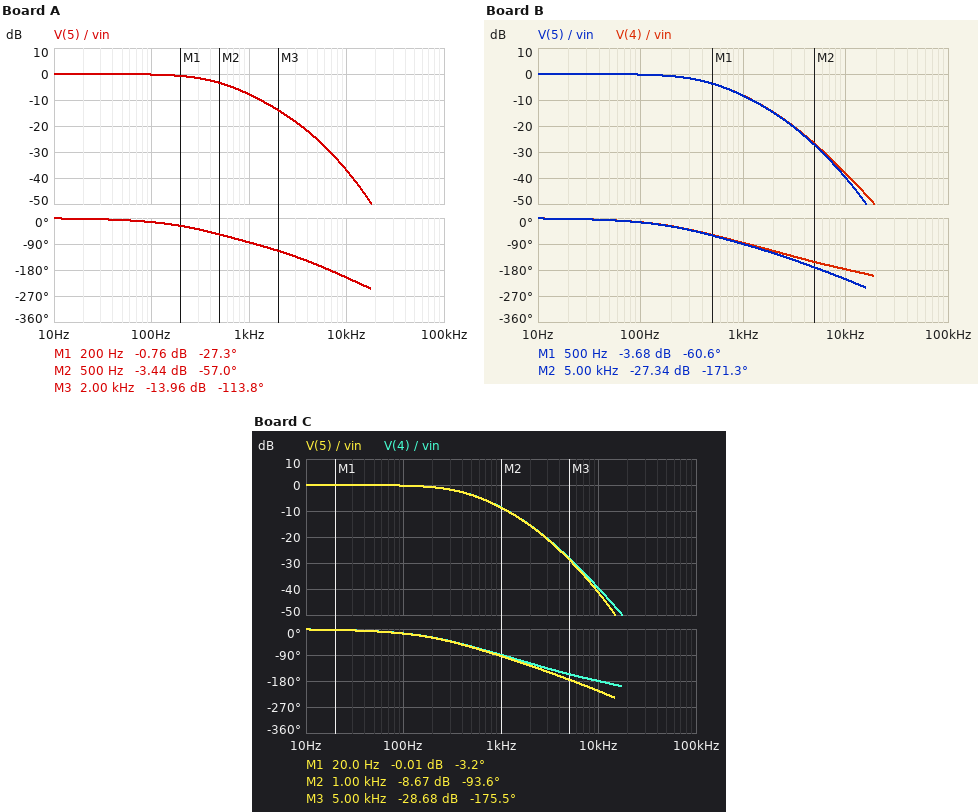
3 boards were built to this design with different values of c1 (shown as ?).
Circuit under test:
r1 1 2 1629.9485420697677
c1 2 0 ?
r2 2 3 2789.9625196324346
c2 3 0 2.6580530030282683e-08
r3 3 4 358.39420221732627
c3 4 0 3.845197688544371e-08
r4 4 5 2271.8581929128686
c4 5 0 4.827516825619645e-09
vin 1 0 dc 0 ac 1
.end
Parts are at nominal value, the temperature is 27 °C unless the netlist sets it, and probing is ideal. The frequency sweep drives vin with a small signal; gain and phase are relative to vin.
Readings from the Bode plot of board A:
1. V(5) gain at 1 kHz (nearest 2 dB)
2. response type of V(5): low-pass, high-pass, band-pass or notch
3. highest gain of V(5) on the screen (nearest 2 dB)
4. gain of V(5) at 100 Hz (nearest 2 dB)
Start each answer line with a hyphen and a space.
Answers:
- -8 dB
- low-pass
- 0 dB
- 0 dB
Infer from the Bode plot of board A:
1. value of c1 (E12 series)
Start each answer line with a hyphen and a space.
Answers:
- 39 nF
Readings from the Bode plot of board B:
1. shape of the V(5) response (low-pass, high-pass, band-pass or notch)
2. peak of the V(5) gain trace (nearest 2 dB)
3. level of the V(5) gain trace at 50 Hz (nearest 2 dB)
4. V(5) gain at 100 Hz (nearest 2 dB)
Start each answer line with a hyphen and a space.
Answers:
- low-pass
- 0 dB
- 0 dB
- 0 dB
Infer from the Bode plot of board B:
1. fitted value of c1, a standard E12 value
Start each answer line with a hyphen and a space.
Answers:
- 56 nF
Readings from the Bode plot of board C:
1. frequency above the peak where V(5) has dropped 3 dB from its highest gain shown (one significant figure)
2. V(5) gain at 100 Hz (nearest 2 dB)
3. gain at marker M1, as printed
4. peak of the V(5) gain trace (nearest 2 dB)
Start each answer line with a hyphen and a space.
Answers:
- 400 Hz
- 0 dB
- -0.01 dB
- 0 dB
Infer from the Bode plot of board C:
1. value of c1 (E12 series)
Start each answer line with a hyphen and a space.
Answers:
- 68 nF
